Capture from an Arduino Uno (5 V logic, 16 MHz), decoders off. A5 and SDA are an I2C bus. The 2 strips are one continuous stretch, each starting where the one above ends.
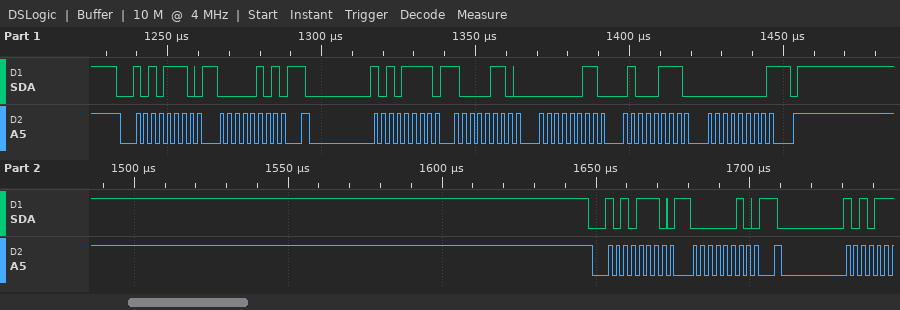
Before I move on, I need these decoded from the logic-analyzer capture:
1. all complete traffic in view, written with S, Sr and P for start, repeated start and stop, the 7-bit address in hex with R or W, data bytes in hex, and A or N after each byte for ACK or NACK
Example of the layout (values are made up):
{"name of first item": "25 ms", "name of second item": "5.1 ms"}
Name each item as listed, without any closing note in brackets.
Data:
{"all complete traffic in view, written with S, Sr and P for start, repeated start and stop, the 7-bit address in hex with R or W, data bytes in hex, and A or N after each byte for ACK or NACK": "S 57W A 05 A Sr 57R A 86 A 03 A 47 A 00 N P S 57W A 02 A"}
